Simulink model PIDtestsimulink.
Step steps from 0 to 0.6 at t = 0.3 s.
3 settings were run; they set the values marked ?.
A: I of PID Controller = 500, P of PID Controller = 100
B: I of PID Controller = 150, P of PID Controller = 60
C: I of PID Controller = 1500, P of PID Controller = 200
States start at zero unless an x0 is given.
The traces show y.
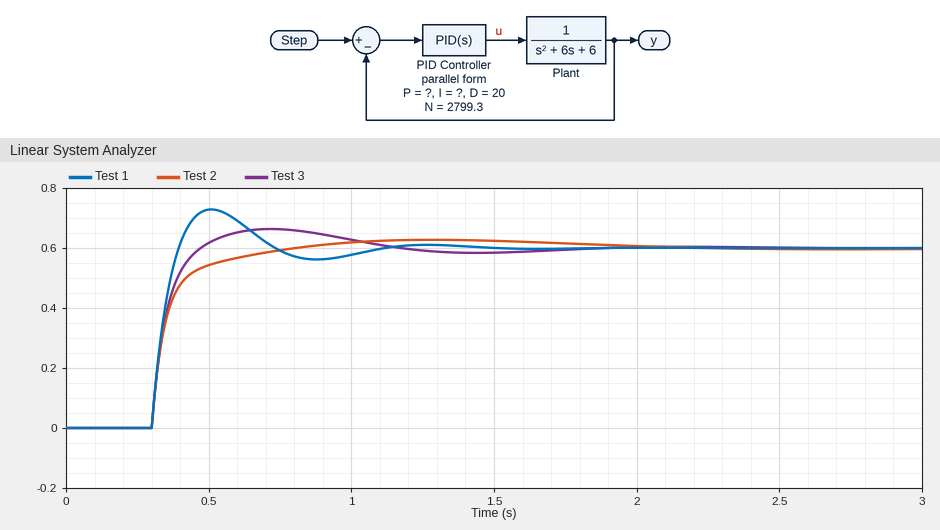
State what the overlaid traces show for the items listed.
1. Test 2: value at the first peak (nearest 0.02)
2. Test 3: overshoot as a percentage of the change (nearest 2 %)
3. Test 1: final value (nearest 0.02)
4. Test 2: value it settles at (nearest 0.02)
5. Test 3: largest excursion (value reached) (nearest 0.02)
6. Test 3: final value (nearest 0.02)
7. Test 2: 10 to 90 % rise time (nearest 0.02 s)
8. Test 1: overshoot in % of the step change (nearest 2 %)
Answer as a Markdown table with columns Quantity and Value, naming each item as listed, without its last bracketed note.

| Quantity | Value |
|---|---|
| Test 2: value at the first peak | 0.62 |
| Test 3: overshoot as a percentage of the change | 10 % |
| Test 1: final value | 0.60 |
| Test 2: value it settles at | 0.60 |
| Test 3: largest excursion (value reached) | 0.66 |
| Test 3: final value | 0.60 |
| Test 2: 10 to 90 % rise time | 0.18 s |
| Test 1: overshoot in % of the step change | 22 % |
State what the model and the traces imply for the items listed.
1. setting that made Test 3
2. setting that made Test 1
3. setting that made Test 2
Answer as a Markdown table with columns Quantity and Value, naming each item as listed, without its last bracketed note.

| Quantity | Value |
|---|---|
| setting that made Test 3 | A |
| setting that made Test 1 | C |
| setting that made Test 2 | B |
